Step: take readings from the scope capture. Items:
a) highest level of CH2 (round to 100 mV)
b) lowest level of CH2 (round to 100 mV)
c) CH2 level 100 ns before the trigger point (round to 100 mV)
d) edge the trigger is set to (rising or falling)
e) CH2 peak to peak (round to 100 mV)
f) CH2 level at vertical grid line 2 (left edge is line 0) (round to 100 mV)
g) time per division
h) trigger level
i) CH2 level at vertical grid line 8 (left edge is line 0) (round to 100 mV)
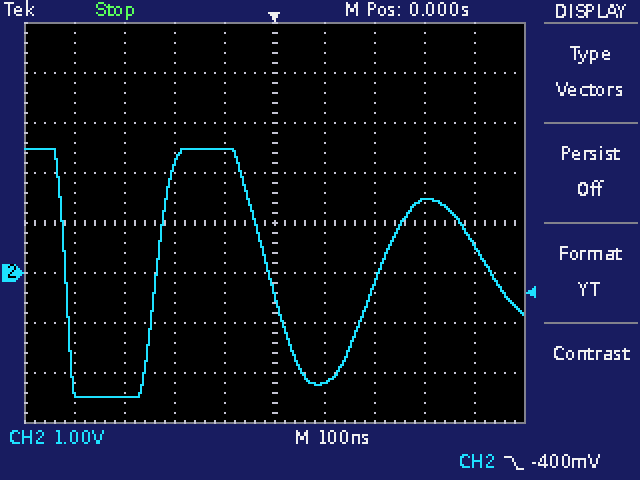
2.5 V
-2.5 V
2.5 V
falling
5.0 V
-2.5 V
100 ns
-400 mV
1.5 V
